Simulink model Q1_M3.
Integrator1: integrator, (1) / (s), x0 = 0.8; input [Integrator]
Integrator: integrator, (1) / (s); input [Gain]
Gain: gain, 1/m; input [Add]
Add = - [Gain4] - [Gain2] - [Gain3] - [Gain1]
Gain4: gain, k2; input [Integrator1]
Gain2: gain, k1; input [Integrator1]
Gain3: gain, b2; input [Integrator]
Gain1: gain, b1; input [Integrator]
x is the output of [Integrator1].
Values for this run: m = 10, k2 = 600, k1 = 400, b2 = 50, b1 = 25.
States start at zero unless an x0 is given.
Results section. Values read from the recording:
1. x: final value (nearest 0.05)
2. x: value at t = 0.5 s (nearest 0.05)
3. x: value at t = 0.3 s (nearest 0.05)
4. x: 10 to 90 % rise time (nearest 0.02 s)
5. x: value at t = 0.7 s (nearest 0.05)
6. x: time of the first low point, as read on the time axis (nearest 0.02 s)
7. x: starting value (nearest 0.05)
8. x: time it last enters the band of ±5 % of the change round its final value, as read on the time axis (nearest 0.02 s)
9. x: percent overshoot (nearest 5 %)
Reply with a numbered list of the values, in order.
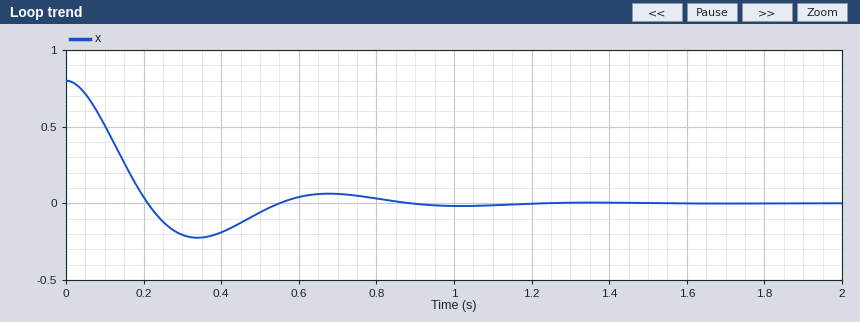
1. 0.00
2. -0.05
3. -0.20
4. 0.14 s
5. 0.05
6. 0.34 s
7. 0.80
8. 0.78 s
9. 30 %
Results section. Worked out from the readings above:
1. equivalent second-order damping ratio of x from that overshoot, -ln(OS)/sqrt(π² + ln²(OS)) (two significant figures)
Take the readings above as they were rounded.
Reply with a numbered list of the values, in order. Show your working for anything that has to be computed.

1. ln(0.3) = -1.204; 1.204 / sqrt(9.870 + 1.450) = 0.36
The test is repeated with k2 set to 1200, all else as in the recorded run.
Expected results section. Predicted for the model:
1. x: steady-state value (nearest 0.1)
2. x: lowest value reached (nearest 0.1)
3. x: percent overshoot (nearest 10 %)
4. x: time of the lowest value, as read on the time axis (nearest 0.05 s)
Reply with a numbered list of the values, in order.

1. 0.0
2. -0.3
3. 40 %
4. 0.25 s
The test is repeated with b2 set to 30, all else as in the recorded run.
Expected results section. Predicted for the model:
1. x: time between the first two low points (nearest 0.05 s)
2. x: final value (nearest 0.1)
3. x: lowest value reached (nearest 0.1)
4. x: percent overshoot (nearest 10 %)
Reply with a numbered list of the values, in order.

1. 0.65 s
2. 0.0
3. -0.3
4. 40 %
